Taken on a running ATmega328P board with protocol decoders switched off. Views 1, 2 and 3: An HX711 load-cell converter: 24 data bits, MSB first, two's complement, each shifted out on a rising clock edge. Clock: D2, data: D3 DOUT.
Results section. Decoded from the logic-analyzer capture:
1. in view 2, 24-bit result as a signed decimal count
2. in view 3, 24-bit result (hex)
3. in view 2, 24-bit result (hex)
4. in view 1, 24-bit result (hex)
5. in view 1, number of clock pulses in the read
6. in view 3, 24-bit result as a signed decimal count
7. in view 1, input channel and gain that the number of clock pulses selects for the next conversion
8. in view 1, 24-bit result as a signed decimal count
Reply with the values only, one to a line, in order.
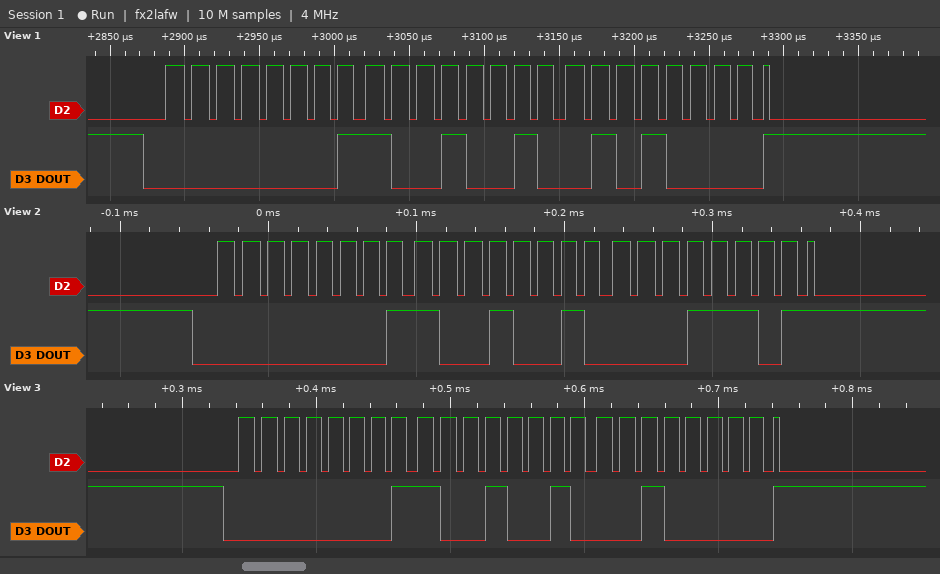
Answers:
102941
0x019220
0x01921D
0x019250
25
102944
channel A, gain 128
102992
